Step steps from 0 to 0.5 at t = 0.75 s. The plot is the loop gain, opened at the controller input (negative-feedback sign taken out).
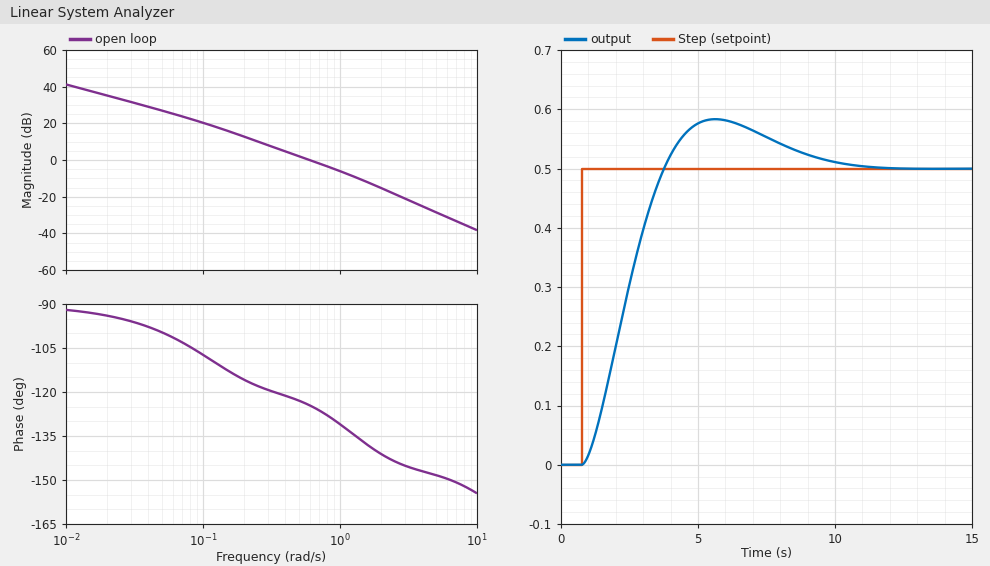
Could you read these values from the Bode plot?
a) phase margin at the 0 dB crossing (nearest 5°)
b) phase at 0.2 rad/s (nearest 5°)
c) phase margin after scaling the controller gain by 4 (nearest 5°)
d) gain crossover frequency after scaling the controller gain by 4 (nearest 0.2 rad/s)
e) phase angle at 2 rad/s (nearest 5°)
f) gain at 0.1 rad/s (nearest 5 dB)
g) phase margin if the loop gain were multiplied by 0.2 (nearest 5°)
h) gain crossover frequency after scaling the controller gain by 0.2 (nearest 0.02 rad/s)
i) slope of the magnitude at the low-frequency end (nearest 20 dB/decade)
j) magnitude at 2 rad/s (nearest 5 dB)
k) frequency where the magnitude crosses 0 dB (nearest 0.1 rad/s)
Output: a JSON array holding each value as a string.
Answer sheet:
["55°", "-115°", "40°", "1.6 rad/s", "-140°", "20 dB", "65°", "0.18 rad/s", "-20 dB/decade", "-15 dB", "0.6 rad/s"]
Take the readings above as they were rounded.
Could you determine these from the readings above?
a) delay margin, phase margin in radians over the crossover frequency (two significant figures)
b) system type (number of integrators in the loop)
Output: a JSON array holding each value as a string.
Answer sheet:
["1.6 s", "1"]
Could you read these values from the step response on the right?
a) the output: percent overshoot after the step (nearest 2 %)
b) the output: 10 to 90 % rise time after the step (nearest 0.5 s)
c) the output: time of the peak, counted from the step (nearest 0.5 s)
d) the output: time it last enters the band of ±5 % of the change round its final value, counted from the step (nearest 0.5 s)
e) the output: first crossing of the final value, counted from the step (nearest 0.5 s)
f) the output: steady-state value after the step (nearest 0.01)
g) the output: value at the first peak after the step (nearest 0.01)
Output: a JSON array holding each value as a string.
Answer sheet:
["16 %", "2.0 s", "5.0 s", "8.0 s", "3.0 s", "0.50", "0.58"]
